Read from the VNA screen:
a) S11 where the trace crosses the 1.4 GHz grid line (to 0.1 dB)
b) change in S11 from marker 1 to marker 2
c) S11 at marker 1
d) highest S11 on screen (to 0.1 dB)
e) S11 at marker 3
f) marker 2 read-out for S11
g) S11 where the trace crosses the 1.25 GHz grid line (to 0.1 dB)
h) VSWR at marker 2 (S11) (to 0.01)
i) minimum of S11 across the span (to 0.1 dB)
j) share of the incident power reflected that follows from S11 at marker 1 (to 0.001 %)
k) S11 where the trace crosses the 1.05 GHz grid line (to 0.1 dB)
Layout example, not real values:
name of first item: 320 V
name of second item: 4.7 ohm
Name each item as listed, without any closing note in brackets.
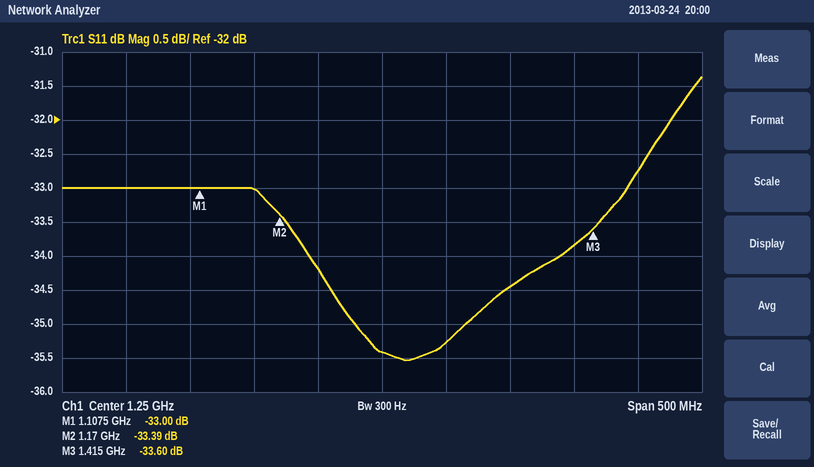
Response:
S11 where the trace crosses the 1.4 GHz grid line: -33.8 dB
change in S11 from marker 1 to marker 2: -0.39 dB
S11 at marker 1: -33.00 dB
highest S11 on screen: -31.4 dB
S11 at marker 3: -33.60 dB
marker 2 read-out for S11: -33.39 dB
S11 where the trace crosses the 1.25 GHz grid line: -35.4 dB
VSWR at marker 2 (S11): 1.04
minimum of S11 across the span: -35.5 dB
share of the incident power reflected that follows from S11 at marker 1: 0.050 %
S11 where the trace crosses the 1.05 GHz grid line: -33.0 dB
